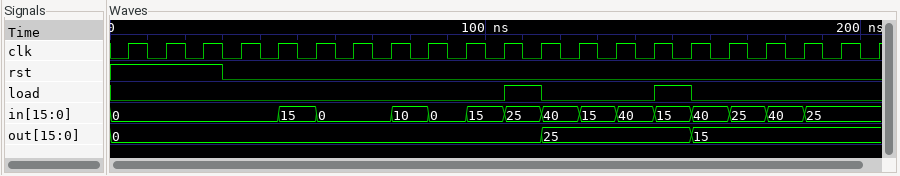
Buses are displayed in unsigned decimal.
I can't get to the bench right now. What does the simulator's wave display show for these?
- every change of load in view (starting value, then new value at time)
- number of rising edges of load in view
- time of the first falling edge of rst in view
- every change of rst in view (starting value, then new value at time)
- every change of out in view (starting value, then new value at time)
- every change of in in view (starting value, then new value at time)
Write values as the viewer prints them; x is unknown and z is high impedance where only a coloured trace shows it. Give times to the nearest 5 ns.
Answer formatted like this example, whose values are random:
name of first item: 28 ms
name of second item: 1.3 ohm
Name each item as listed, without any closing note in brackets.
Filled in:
every change of load in view: 0, 1 at 105 ns, 0 at 115 ns, 1 at 145 ns, 0 at 155 ns
number of rising edges of load in view: 2
time of the first falling edge of rst in view: 30 ns
every change of rst in view: 1, 0 at 30 ns
every change of out in view: 0, 25 at 115 ns, 15 at 155 ns
every change of in in view: 0, 15 at 45 ns, 0 at 55 ns, 10 at 75 ns, 0 at 85 ns, 15 at 95 ns, 25 at 105 ns, 40 at 115 ns, 15 at 125 ns, 40 at 135 ns, 15 at 145 ns, 40 at 155 ns, 25 at 165 ns, 40 at 175 ns, 25 at 185 ns
